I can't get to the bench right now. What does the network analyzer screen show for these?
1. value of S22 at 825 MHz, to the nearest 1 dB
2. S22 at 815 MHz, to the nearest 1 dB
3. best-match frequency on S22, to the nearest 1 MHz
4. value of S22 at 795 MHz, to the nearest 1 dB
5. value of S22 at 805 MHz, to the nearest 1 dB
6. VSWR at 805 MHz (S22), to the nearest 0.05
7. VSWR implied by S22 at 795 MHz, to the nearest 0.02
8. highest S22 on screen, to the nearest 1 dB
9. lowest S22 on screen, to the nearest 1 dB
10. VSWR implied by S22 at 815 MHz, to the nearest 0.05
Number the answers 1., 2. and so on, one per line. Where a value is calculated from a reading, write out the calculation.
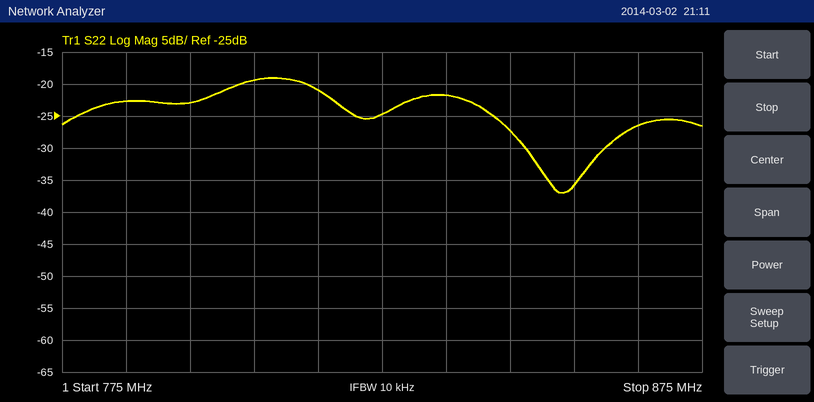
1. -25 dB
2. -21 dB
3. 853 MHz
4. -23 dB
5. -19 dB
6. |Γ| = 10^(-19/20) = 0.1122; VSWR = (1 + 0.1122)/(1 − 0.1122) ≈ 1.25
7. |Γ| = 10^(-23/20) = 0.0708; VSWR = (1 + 0.0708)/(1 − 0.0708) ≈ 1.15, so 1.16 to the nearest 0.02
8. -19 dB
9. -37 dB
10. |Γ| = 10^(-21/20) = 0.0891; VSWR = (1 + 0.0891)/(1 − 0.0891) ≈ 1.20
